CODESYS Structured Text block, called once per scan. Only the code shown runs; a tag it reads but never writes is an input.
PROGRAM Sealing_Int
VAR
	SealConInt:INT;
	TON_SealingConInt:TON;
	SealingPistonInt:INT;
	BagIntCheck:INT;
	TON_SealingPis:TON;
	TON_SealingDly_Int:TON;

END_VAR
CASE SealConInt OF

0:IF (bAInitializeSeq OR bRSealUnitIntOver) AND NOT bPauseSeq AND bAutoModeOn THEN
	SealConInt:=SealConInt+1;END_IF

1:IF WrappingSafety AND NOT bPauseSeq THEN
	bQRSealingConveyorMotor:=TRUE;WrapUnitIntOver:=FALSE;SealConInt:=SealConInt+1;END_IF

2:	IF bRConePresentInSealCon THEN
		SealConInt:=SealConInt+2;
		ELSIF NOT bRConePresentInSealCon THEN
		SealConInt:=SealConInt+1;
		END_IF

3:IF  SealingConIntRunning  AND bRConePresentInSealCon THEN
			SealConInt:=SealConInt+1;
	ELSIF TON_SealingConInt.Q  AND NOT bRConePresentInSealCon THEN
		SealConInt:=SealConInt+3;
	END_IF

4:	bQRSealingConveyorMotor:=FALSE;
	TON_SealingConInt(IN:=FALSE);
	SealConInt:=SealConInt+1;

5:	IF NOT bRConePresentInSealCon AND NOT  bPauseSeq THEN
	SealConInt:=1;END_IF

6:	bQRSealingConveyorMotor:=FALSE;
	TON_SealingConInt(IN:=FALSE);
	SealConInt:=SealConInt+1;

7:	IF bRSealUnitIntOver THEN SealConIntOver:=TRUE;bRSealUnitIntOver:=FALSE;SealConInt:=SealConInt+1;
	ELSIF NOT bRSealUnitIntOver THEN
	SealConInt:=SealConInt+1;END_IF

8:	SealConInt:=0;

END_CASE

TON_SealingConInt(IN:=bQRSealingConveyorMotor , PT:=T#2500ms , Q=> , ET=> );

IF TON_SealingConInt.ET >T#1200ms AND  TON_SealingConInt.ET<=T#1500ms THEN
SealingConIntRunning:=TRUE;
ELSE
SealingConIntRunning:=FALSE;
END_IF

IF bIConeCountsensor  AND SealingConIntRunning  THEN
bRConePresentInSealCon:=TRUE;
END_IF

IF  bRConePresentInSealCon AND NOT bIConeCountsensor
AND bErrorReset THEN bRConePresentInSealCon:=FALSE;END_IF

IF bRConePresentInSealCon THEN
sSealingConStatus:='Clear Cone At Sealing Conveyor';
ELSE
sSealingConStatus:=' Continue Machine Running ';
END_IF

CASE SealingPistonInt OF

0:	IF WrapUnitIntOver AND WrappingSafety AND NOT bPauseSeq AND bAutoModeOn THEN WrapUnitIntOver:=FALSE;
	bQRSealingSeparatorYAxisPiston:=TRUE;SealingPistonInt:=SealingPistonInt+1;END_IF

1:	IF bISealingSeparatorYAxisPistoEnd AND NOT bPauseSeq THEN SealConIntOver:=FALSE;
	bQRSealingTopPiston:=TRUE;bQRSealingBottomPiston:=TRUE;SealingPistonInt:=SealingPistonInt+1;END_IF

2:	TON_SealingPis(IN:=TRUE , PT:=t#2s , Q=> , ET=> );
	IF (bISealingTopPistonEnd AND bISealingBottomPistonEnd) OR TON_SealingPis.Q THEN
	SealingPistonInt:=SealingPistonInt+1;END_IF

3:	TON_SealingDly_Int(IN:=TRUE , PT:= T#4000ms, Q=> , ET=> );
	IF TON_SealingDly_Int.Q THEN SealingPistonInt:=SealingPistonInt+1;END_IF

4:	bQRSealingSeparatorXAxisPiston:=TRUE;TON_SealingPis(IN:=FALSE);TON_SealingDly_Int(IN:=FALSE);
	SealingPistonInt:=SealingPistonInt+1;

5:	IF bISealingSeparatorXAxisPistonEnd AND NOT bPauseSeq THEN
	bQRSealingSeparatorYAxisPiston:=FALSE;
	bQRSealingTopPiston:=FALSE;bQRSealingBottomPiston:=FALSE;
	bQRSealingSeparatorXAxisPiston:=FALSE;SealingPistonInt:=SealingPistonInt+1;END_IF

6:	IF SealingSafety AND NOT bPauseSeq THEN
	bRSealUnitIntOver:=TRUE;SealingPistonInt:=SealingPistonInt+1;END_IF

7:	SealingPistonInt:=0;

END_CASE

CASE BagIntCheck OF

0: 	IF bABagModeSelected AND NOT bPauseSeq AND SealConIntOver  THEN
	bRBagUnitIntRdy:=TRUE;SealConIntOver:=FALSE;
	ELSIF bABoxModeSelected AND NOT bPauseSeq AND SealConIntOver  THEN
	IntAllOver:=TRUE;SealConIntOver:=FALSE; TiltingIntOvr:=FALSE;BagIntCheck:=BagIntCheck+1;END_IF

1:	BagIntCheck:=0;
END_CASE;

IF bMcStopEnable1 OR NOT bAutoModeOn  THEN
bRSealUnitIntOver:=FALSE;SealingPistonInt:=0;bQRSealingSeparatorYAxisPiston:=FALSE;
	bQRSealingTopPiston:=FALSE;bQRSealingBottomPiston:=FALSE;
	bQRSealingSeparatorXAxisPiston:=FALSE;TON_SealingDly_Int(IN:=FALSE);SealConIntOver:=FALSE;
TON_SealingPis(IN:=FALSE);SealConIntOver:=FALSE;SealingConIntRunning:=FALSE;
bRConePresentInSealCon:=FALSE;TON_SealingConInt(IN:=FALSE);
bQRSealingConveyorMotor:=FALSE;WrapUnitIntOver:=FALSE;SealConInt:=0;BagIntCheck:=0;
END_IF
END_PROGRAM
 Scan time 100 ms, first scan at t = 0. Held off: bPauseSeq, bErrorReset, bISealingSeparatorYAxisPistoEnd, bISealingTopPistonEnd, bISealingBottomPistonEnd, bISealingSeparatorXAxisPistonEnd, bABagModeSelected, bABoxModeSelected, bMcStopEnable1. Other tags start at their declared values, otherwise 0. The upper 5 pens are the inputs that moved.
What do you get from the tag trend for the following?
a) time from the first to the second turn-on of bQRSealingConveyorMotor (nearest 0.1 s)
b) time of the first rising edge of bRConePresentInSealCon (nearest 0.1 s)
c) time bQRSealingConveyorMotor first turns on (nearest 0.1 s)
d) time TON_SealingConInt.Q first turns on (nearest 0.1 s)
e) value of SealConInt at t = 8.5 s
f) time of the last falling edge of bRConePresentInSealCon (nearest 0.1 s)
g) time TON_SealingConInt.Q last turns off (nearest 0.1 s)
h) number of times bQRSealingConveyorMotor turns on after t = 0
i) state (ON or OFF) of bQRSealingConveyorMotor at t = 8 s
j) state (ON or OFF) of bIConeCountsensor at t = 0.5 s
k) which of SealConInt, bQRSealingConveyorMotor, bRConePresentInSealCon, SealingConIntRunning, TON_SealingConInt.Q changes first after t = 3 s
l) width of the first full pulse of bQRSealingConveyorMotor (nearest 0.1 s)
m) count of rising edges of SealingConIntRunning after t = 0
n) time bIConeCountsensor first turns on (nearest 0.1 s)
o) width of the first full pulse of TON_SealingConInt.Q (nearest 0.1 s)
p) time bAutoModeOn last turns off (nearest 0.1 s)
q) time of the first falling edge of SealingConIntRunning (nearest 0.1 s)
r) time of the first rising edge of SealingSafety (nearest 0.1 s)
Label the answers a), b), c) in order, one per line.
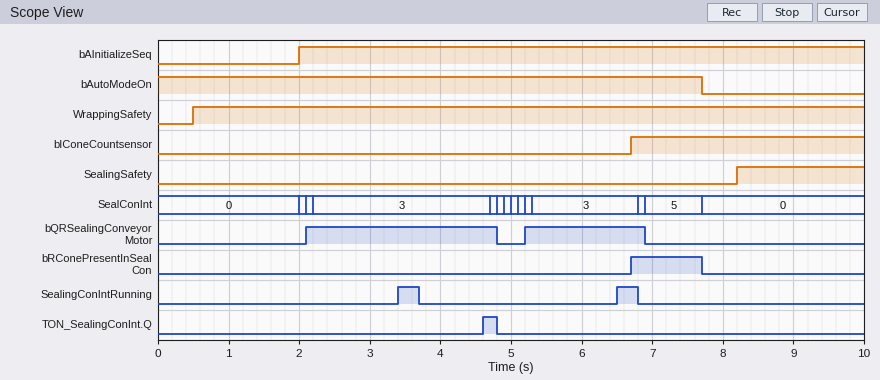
a) 3.1 s
b) 6.7 s
c) 2.1 s
d) 4.6 s
e) 0
f) 7.7 s
g) 4.8 s
h) 2
i) OFF
j) OFF
k) SealingConIntRunning
l) 2.7 s
m) 2
n) 6.7 s
o) 0.2 s
p) 7.7 s
q) 3.7 s
r) 8.2 s
